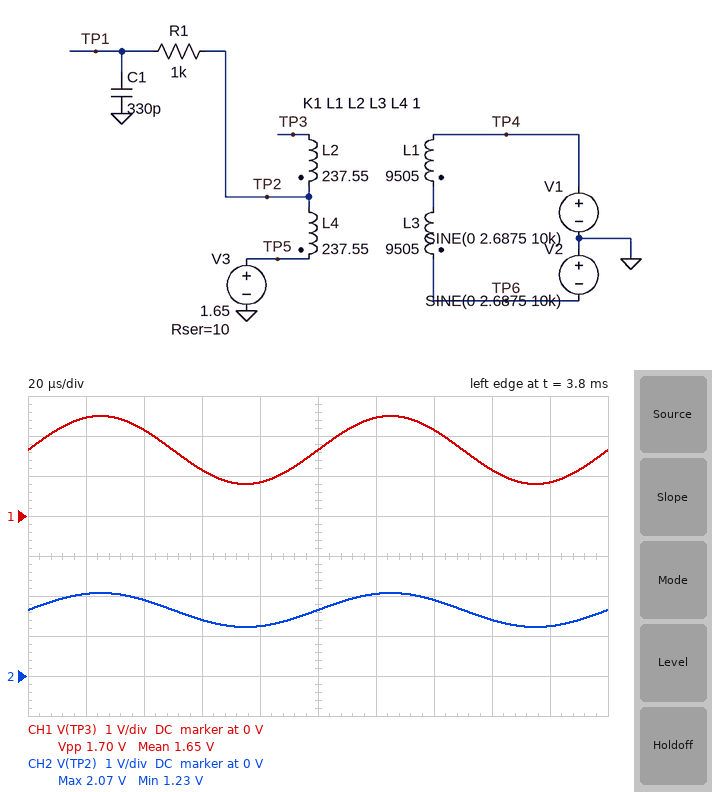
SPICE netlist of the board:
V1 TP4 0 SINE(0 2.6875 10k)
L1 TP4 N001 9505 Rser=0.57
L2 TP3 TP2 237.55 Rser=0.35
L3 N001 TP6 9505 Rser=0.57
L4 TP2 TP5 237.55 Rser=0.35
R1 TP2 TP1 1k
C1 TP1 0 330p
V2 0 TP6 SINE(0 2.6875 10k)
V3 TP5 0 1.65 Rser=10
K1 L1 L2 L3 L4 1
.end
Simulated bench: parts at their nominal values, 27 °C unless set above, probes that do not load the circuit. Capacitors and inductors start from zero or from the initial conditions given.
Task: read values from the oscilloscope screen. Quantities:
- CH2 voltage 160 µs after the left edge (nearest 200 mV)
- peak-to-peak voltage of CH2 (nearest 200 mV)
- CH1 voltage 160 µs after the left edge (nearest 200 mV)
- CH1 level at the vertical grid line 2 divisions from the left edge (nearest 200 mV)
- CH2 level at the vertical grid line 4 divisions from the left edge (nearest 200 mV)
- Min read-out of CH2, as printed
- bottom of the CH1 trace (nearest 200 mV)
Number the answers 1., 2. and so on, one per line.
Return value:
1. 1.4 V
2. 800 mV
3. 1.2 V
4. 2.2 V
5. 1.2 V
6. 1.23 V
7. 800 mV
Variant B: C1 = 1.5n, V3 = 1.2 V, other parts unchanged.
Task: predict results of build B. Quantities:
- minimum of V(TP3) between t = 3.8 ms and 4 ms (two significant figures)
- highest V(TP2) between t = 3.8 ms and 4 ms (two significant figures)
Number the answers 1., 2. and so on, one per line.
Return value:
1. 350 mV
2. 1.6 V
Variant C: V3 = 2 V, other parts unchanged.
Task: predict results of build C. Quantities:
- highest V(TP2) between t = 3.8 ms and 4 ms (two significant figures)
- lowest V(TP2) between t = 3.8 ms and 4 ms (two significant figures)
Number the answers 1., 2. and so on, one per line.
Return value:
1. 2.4 V
2. 1.6 V
